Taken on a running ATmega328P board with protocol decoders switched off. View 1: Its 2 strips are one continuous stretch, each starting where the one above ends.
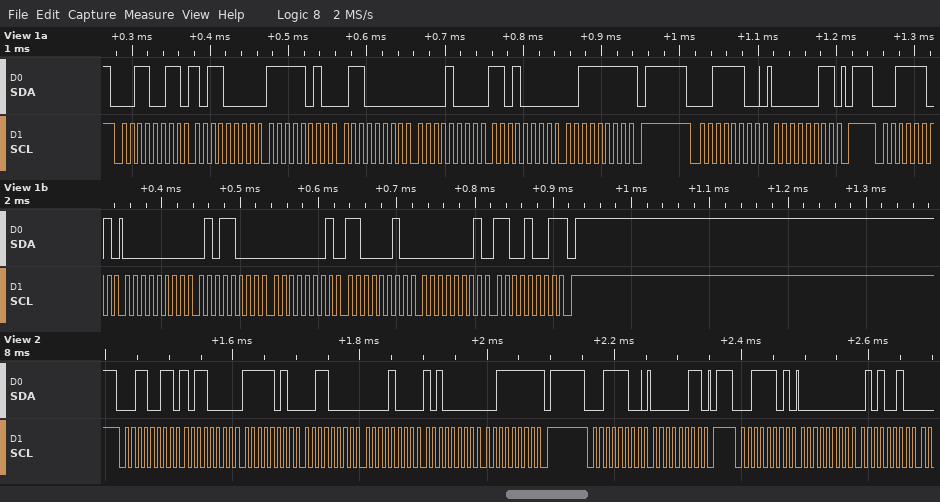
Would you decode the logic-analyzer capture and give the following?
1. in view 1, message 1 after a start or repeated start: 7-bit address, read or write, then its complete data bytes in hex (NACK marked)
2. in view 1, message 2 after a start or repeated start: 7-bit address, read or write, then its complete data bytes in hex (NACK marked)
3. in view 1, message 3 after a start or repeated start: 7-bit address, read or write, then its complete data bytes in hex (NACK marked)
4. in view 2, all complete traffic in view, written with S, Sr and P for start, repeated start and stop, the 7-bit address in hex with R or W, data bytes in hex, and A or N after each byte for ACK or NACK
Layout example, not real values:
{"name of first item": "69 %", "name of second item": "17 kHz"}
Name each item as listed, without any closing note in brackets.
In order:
{"in view 1, message 1 after a start or repeated start: 7-bit address, read or write, then its complete data bytes in hex": "0x19 read: B0 FA 60 08 D0 3F NACK", "in view 1, message 2 after a start or repeated start: 7-bit address, read or write, then its complete data bytes in hex": "0x1E write: 03", "in view 1, message 3 after a start or repeated start: 7-bit address, read or write, then its complete data bytes in hex": "0x1E read: 00 58 01 C2 01 C9 NACK", "in view 2, all complete traffic in view, written with S, Sr and P for start, repeated start and stop, the 7-bit address in hex with R or W, data bytes in hex, and A or N after each byte for ACK or NACK": "S 19R A B0 A FA A 30 A 08 A A0 A 3F N P S 1EW A 03 A P S 1ER A 00 A 52 A"}
